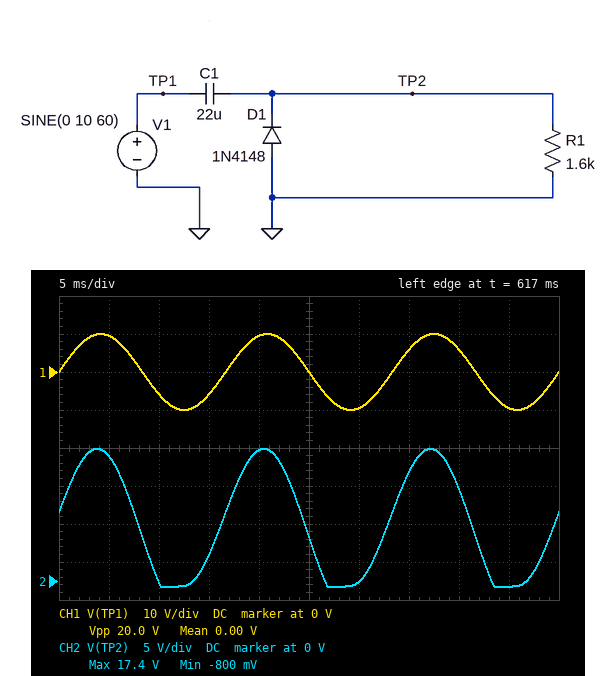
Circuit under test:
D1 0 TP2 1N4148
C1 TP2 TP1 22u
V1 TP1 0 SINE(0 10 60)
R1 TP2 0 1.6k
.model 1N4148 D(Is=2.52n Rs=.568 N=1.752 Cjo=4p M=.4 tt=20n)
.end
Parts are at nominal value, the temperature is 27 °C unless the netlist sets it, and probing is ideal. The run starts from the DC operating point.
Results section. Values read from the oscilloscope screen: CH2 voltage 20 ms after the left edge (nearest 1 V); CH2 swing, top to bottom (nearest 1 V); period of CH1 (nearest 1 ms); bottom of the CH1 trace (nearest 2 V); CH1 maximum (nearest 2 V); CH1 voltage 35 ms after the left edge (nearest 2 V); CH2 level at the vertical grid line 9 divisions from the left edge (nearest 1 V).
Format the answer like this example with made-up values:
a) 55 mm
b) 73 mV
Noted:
a) 17 V
b) 18 V
c) 17 ms
d) -10 V
e) 10 V
f) 6 V
g) -1 V
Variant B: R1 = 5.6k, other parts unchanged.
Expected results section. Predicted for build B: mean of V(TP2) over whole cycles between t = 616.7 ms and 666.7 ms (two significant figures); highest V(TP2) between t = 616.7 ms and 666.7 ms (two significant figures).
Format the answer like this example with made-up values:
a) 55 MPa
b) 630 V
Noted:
a) 8.8 V
b) 19 V
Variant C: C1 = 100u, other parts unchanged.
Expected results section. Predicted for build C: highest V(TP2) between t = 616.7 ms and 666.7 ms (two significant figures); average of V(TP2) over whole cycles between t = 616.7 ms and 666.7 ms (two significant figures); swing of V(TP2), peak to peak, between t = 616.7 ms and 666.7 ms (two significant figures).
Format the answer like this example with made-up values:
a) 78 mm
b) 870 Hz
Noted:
a) 19 V
b) 8.9 V
c) 20 V
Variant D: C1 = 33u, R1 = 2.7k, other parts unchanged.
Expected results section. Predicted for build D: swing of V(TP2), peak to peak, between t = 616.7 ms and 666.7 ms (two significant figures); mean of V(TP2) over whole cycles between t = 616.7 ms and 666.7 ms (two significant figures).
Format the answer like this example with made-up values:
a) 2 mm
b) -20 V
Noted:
a) 19 V
b) 8.6 V
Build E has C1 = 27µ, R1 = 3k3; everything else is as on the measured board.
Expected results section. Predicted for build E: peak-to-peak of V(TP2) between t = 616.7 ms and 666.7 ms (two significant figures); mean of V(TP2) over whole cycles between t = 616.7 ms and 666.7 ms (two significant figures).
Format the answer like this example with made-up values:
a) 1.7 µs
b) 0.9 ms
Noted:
a) 19 V
b) 8.6 V
